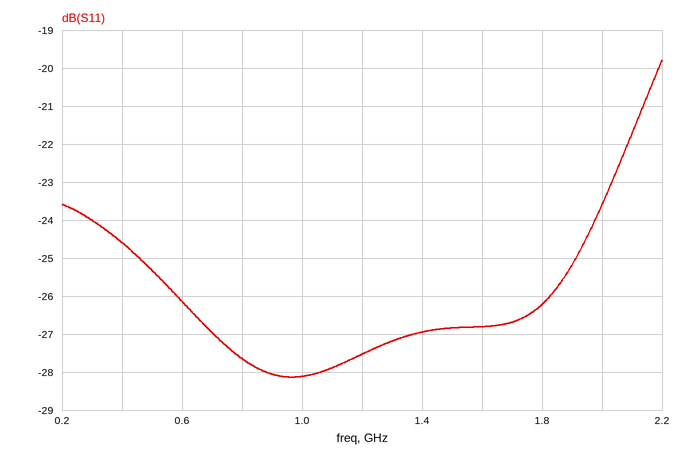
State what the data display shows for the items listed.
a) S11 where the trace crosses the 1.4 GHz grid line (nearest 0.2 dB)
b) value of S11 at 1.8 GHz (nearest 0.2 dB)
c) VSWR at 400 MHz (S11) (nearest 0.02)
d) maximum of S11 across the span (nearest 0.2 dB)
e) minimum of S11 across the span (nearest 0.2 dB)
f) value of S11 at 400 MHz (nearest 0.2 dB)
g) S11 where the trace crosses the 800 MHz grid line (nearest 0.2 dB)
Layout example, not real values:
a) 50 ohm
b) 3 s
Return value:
a) -27.0 dB
b) -26.2 dB
c) 1.12
d) -19.8 dB
e) -28.2 dB
f) -24.6 dB
g) -27.6 dB
